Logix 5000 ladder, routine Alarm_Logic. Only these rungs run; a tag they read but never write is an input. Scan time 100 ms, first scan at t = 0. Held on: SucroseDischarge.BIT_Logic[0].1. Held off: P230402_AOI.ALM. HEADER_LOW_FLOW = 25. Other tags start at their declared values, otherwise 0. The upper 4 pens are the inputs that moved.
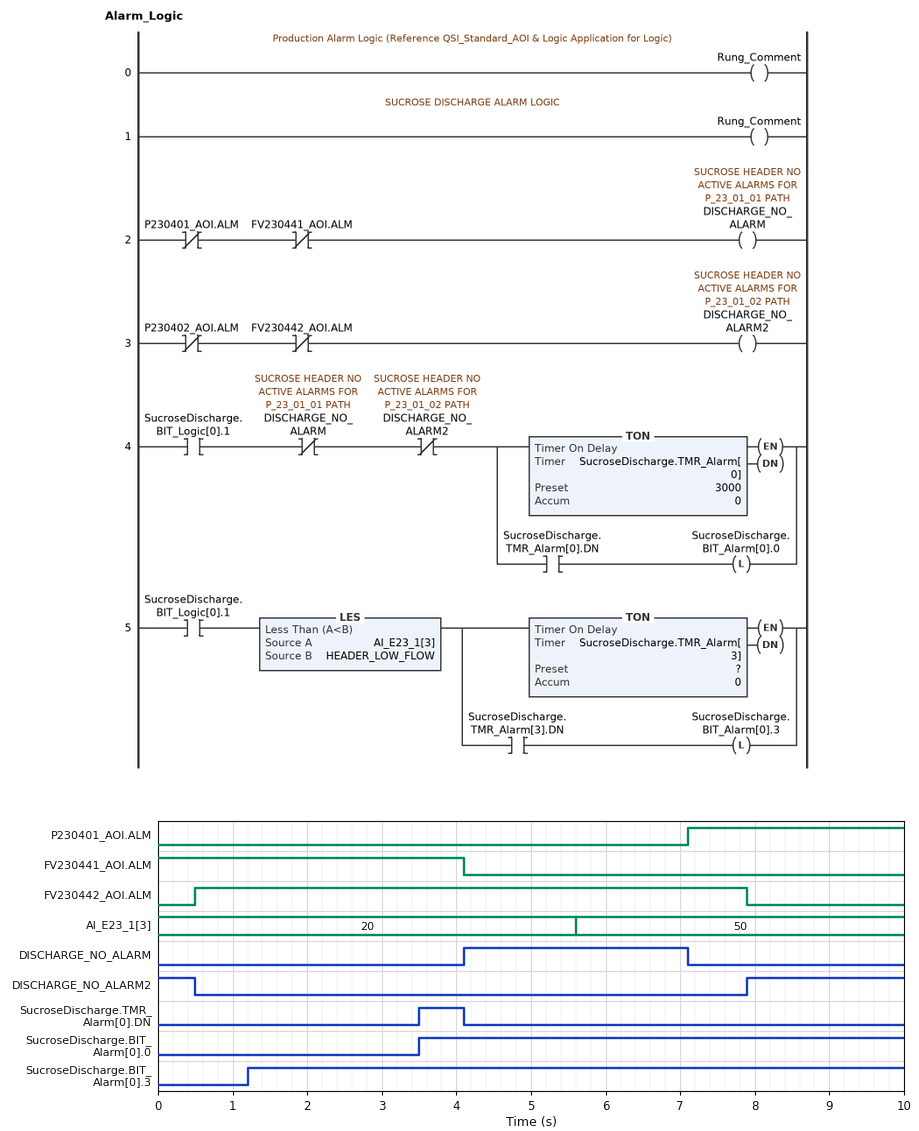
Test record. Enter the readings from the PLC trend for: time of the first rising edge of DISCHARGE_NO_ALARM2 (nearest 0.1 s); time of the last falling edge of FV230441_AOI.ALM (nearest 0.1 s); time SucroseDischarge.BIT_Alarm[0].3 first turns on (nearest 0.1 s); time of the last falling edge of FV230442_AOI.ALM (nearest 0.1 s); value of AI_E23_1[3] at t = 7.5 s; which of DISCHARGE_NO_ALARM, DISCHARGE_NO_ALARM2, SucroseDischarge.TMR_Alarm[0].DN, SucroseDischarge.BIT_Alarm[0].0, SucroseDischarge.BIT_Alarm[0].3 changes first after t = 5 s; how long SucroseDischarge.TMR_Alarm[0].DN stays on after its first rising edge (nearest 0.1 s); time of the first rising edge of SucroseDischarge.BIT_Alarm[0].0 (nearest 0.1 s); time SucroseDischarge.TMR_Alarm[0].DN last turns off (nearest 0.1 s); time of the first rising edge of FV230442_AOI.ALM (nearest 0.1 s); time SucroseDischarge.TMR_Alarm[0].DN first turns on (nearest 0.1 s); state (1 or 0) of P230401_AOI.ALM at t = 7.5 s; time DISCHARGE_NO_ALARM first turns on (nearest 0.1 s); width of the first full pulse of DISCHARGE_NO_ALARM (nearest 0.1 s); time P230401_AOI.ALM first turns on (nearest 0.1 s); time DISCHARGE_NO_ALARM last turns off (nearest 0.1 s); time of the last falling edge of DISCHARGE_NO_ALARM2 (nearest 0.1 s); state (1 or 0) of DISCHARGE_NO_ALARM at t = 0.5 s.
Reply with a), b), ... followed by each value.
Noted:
a) 7.9 s
b) 4.1 s
c) 1.2 s
d) 7.9 s
e) 50
f) DISCHARGE_NO_ALARM
g) 0.6 s
h) 3.5 s
i) 4.1 s
j) 0.5 s
k) 3.5 s
l) 1
m) 4.1 s
n) 3.0 s
o) 7.1 s
p) 7.1 s
q) 0.5 s
r) 0
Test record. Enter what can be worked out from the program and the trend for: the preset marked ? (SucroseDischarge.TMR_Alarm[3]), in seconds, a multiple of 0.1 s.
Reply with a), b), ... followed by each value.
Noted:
a) 1.2 s
